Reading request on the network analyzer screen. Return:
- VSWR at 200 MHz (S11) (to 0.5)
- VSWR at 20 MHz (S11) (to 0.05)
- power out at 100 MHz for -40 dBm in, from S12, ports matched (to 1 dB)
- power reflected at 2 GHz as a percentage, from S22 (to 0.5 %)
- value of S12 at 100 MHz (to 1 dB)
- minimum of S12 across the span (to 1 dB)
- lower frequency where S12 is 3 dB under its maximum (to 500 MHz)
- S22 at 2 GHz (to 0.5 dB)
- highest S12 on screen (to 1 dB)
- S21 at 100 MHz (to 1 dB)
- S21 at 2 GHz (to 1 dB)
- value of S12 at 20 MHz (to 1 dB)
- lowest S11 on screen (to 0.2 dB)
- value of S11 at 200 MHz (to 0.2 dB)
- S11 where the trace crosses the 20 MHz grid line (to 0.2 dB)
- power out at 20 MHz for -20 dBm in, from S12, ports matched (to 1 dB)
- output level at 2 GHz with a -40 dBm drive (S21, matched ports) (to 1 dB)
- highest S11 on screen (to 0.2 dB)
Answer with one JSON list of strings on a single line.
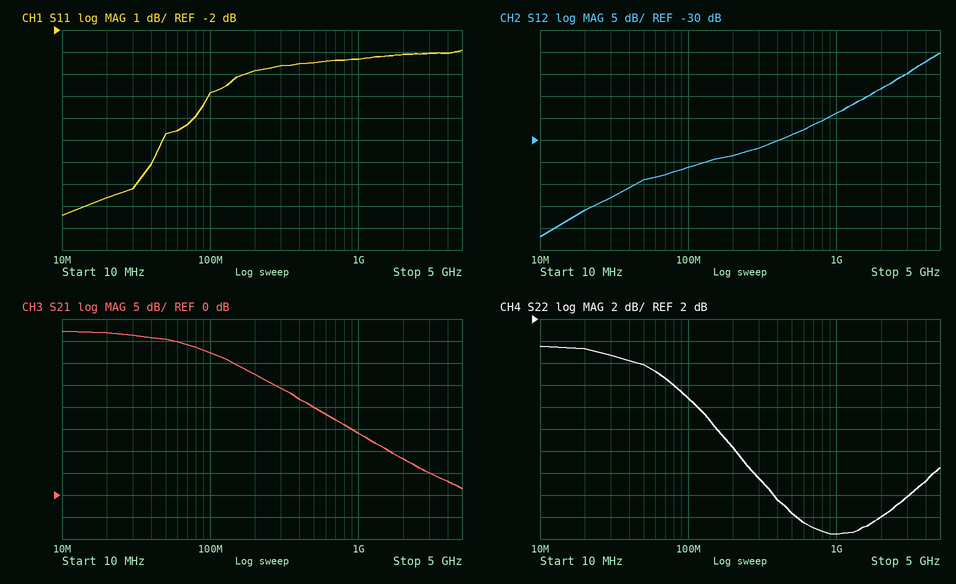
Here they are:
["4.5", "2.00", "-76 dBm", "2.5 %", "-36 dB", "-52 dB", "3.5 GHz", "-16.0 dB", "-10 dB", "32 dB", "8 dB", "-46 dB", "-10.4 dB", "-3.8 dB", "-9.6 dB", "-66 dBm", "-32 dBm", "-3.0 dB"]
